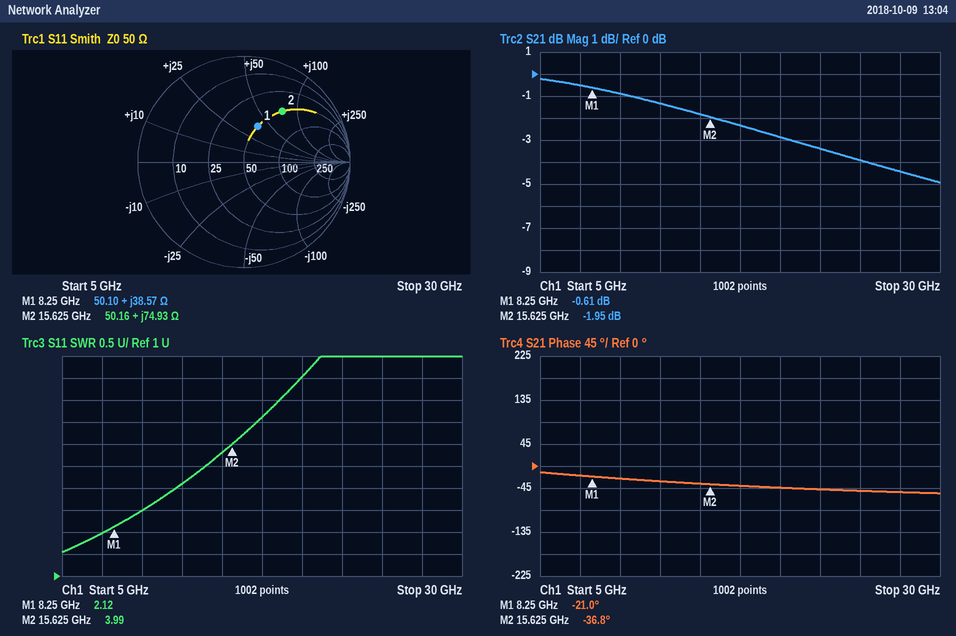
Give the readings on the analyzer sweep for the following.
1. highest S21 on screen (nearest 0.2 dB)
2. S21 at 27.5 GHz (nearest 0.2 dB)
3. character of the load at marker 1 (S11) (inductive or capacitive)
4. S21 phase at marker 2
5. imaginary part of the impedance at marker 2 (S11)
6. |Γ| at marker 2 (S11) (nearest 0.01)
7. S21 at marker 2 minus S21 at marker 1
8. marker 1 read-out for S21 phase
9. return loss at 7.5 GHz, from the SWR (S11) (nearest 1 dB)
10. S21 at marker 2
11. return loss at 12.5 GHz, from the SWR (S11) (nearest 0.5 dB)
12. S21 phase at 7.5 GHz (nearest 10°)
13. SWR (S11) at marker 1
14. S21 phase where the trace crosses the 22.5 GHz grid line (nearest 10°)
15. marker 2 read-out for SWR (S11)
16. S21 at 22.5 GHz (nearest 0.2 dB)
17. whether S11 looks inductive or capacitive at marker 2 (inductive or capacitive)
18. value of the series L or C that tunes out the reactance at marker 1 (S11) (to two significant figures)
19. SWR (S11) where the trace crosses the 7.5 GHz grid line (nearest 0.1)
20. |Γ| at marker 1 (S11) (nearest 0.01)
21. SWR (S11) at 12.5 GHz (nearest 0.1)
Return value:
-0.2 dB
-4.4 dB
inductive
-36.8°
+74.93 Ω
0.60
-1.34 dB
-21.0°
10 dB
-1.95 dB
6.0 dB
-20°
2.12
-50°
3.99
-3.4 dB
inductive
500 fF
2.0
0.36
3.1
